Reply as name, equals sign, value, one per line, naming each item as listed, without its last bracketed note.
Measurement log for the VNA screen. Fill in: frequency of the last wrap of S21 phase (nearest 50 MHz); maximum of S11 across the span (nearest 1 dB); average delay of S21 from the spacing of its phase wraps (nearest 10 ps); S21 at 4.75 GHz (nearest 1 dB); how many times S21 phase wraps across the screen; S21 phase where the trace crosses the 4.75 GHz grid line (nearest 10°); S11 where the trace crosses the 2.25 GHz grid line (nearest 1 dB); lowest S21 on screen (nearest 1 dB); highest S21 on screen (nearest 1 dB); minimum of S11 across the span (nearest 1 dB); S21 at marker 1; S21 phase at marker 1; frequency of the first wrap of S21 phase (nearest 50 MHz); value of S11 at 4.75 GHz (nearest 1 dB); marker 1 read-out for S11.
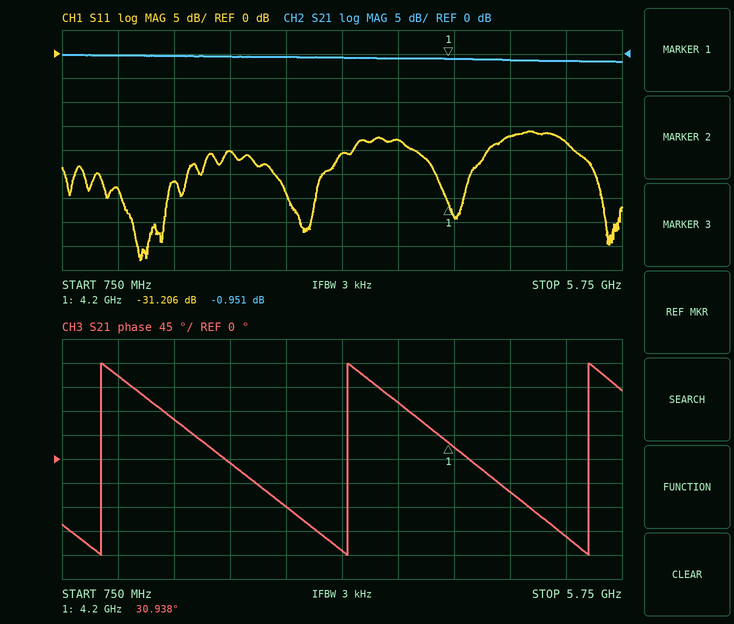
frequency of the last wrap of S21 phase = 5.45 GHz
maximum of S11 across the span = -16 dB
average delay of S21 from the spacing of its phase wraps = 460 ps
S21 at 4.75 GHz = -1 dB
how many times S21 phase wraps across the screen = 3
S21 phase where the trace crosses the 4.75 GHz grid line = -60°
S11 where the trace crosses the 2.25 GHz grid line = -20 dB
lowest S21 on screen = -2 dB
highest S21 on screen = 0 dB
minimum of S11 across the span = -43 dB
S21 at marker 1 = -0.951 dB
S21 phase at marker 1 = 30.938°
frequency of the first wrap of S21 phase = 1.10 GHz
value of S11 at 4.75 GHz = -17 dB
marker 1 read-out for S11 = -31.206 dB
